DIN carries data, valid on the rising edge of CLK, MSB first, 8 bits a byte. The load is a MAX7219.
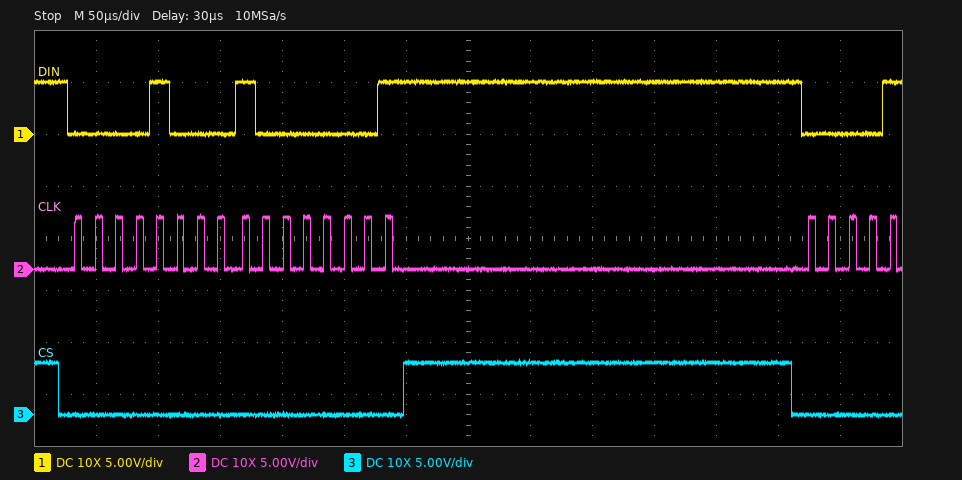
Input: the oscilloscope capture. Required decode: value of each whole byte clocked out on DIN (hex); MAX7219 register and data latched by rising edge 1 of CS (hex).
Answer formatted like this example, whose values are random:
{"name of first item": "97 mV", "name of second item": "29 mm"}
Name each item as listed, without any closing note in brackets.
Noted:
{"value of each whole byte clocked out on DIN": "08 81", "MAX7219 register and data latched by rising edge 1 of CS": "register 0x8, data 0x81"}
